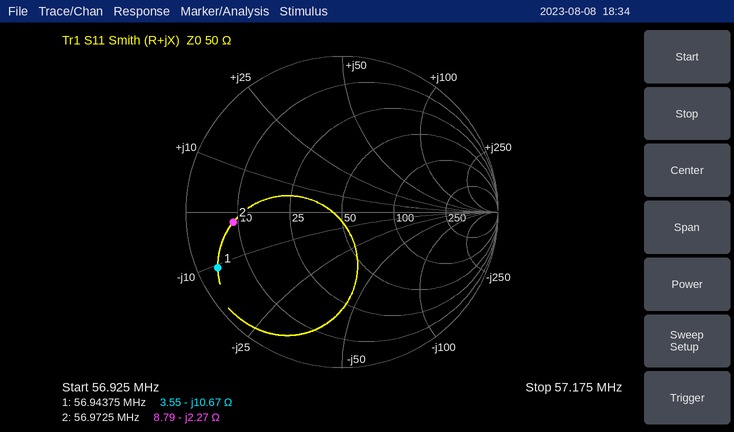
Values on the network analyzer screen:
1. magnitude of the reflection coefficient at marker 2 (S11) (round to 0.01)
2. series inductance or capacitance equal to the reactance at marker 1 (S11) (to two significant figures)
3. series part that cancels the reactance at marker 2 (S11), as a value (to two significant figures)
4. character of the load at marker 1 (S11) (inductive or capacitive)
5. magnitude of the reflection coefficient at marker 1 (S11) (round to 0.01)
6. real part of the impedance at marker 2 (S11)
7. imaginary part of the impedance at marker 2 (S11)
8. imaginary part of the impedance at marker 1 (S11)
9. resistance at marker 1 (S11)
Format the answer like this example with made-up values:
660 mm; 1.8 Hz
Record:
0.70; 260 pF; 6.3 nH; capacitive; 0.87; 8.79 Ω; -2.27 Ω; -10.67 Ω; 3.55 Ω
